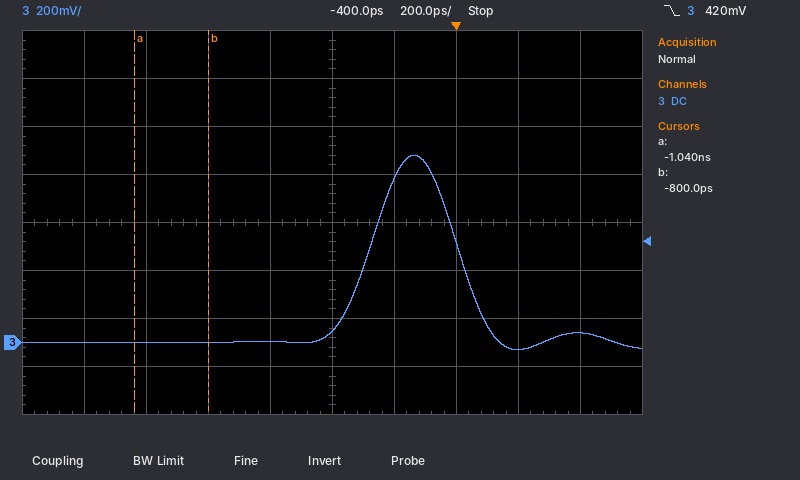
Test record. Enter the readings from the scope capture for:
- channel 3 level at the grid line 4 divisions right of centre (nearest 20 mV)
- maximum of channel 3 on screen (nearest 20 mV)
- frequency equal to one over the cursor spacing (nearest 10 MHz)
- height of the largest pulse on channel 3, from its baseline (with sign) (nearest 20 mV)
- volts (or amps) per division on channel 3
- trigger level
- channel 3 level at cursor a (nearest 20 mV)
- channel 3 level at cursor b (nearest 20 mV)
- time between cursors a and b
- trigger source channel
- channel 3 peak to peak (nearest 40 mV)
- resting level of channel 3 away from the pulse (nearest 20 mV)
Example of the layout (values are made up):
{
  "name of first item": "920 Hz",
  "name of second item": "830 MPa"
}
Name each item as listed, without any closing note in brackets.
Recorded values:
{
  "channel 3 level at the grid line 4 divisions right of centre": "40 mV",
  "maximum of channel 3 on screen": "780 mV",
  "frequency equal to one over the cursor spacing": "4.17 GHz",
  "height of the largest pulse on channel 3, from its baseline (with sign)": "+780 mV",
  "volts (or amps) per division on channel 3": "200 mV",
  "trigger level": "420 mV",
  "channel 3 level at cursor a": "0 mV",
  "channel 3 level at cursor b": "0 mV",
  "time between cursors a and b": "240 ps",
  "trigger source channel": "channel 3",
  "channel 3 peak to peak": "800 mV",
  "resting level of channel 3 away from the pulse": "0 mV"
}
